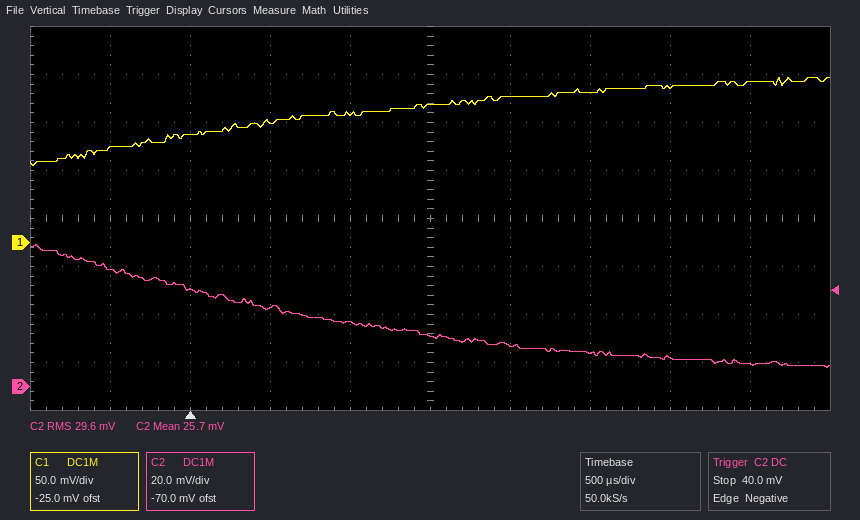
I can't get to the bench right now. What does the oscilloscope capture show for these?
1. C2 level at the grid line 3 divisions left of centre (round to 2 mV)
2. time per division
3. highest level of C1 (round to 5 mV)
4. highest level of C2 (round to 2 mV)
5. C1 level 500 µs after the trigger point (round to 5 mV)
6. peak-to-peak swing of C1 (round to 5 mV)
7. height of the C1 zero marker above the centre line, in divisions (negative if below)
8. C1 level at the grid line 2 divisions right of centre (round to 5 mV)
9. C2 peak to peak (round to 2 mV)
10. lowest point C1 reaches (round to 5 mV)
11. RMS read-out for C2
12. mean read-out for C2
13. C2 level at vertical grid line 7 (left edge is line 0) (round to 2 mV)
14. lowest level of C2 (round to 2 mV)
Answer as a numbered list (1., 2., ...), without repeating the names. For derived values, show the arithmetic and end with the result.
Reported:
1. 40 mV
2. 500 µs
3. 170 mV
4. 60 mV
5. 125 mV
6. 170 mV − (80 mV) = 90 mV
7. -0.5 div
8. 155 mV
9. 60 mV − (8 mV) = 52 mV
10. 80 mV
11. 29.6 mV
12. 25.7 mV
13. 14 mV
14. 8 mV
